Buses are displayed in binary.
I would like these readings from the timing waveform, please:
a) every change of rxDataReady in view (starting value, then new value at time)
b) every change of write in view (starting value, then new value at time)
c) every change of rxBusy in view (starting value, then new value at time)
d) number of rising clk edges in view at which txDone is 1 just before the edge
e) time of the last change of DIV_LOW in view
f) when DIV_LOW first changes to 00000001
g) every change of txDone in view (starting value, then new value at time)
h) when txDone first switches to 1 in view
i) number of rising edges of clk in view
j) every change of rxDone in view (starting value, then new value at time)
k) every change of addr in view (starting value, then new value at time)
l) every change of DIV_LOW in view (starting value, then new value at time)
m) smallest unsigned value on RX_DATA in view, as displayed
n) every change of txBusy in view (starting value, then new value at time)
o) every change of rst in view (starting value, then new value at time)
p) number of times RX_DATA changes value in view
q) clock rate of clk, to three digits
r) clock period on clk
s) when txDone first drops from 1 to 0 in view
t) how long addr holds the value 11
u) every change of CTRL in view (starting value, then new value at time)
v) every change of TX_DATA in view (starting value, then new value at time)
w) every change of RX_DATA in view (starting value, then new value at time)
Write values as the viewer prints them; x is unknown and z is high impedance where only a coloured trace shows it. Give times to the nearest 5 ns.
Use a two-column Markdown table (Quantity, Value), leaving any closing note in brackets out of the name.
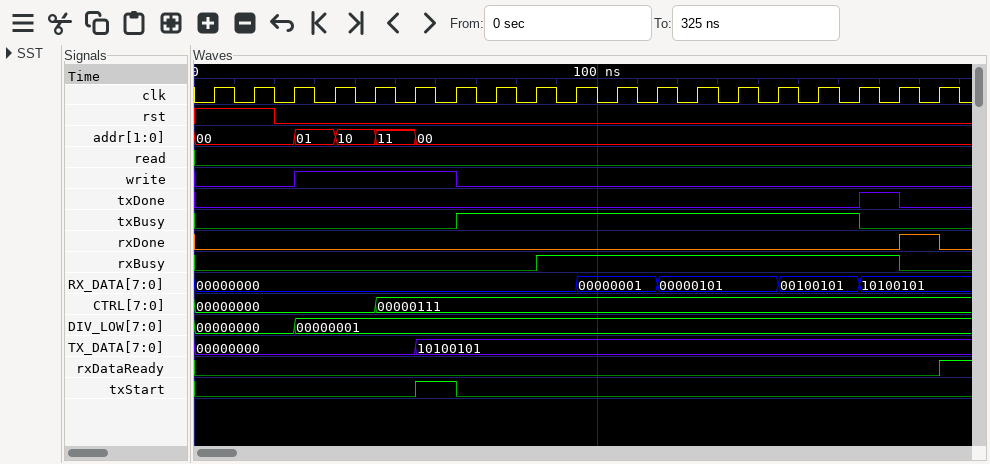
| Quantity | Value |
|---|---|
| every change of rxDataReady in view | 0, 1 at 185 ns |
| every change of write in view | 0, 1 at 25 ns, 0 at 65 ns |
| every change of rxBusy in view | 0, 1 at 85 ns, 0 at 175 ns |
| number of rising clk edges in view at which txDone is 1 just before the edge | 1 |
| time of the last change of DIV_LOW in view | 25 ns |
| when DIV_LOW first changes to 00000001 | 25 ns |
| every change of txDone in view | 0, 1 at 165 ns, 0 at 175 ns |
| when txDone first switches to 1 in view | 165 ns |
| number of rising edges of clk in view | 19 |
| every change of rxDone in view | 0, 1 at 175 ns, 0 at 185 ns |
| every change of addr in view | 00, 01 at 25 ns, 10 at 35 ns, 11 at 45 ns, 00 at 55 ns |
| every change of DIV_LOW in view | 00000000, 00000001 at 25 ns |
| smallest unsigned value on RX_DATA in view, as displayed | 00000000 |
| every change of txBusy in view | 0, 1 at 65 ns, 0 at 165 ns |
| every change of rst in view | 1, 0 at 20 ns |
| number of times RX_DATA changes value in view | 4 |
| clock rate of clk, to three digits | 100 MHz |
| clock period on clk | 10 ns |
| when txDone first drops from 1 to 0 in view | 175 ns |
| how long addr holds the value 11 | 10 ns |
| every change of CTRL in view | 00000000, 00000111 at 45 ns |
| every change of TX_DATA in view | 00000000, 10100101 at 55 ns |
| every change of RX_DATA in view | 00000000, 00000001 at 95 ns, 00000101 at 115 ns, 00100101 at 145 ns, 10100101 at 165 ns |
